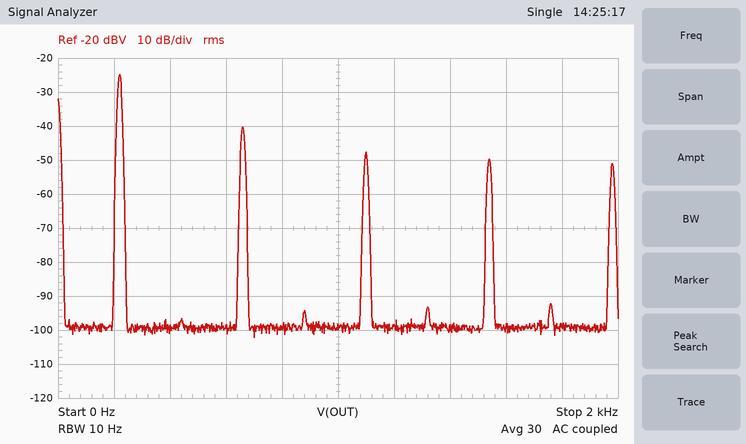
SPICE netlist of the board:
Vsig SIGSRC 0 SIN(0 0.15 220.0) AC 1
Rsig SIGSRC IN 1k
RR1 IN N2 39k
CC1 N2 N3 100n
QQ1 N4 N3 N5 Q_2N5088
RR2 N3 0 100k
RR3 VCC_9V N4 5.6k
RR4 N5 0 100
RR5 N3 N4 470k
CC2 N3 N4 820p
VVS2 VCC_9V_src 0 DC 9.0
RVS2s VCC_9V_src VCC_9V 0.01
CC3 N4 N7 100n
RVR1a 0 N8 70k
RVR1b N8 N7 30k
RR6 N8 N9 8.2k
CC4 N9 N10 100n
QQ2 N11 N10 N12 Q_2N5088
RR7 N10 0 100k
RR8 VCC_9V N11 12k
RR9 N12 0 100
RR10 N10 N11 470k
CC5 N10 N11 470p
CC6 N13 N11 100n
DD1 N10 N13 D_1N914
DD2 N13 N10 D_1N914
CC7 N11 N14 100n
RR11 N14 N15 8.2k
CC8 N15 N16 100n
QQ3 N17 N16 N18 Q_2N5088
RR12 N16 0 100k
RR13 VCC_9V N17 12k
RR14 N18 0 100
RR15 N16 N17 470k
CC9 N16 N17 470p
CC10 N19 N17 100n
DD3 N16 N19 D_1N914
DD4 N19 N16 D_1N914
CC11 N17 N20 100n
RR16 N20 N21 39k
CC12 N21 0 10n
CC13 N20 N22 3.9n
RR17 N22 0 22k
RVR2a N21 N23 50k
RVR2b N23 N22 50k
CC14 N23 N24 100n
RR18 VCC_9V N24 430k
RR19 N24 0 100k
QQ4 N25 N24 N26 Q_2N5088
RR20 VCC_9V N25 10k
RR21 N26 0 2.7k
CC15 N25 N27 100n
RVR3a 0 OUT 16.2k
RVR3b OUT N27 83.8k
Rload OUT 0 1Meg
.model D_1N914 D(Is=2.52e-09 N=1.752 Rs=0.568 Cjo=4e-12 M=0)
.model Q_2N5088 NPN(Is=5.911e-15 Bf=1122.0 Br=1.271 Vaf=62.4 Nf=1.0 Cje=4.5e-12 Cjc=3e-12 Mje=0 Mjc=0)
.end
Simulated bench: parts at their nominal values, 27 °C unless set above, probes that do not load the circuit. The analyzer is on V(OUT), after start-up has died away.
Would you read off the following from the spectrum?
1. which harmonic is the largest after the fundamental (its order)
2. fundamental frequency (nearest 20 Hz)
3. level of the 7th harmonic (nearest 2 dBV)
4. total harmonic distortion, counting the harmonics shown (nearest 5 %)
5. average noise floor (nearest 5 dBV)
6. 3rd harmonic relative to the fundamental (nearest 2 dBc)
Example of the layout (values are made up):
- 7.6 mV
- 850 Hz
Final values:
- 3
- 220 Hz
- -50 dBV
- 20 %
- -100 dBV
- -16 dBc
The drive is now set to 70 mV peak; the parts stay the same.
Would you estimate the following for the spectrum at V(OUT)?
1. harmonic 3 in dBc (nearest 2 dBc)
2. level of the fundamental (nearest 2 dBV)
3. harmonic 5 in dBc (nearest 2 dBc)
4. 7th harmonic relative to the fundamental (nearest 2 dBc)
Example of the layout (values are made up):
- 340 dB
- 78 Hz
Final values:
- -16 dBc
- -26 dBV
- -24 dBc
- -28 dBc
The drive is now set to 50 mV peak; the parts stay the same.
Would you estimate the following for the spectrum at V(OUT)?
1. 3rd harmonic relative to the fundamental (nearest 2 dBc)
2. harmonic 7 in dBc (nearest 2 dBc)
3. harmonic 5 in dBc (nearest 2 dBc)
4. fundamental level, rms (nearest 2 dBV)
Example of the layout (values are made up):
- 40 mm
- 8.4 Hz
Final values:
- -18 dBc
- -28 dBc
- -26 dBc
- -26 dBV
